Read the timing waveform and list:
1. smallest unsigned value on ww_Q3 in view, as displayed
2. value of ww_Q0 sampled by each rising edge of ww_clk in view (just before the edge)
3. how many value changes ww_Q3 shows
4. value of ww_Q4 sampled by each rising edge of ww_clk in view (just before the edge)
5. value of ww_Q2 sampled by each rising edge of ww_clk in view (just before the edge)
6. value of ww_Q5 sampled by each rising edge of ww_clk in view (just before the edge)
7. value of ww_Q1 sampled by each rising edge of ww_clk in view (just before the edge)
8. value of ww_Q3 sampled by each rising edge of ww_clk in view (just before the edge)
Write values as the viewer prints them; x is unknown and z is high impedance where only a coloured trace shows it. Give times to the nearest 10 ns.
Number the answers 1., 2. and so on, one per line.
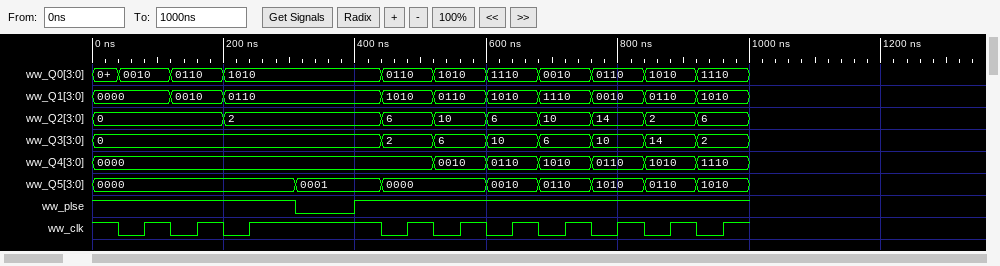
1. 0
2. 0010, 0110, 1010, 0110, 1010, 1110, 0010, 0110, 1010, 1110
3. 7
4. 0000, 0000, 0000, 0000, 0010, 0110, 1010, 0110, 1010, 1110
5. 0, 0, 2, 6, 10, 6, 10, 14, 2, 6
6. 0000, 0000, 0000, 0000, 0000, 0010, 0110, 1010, 0110, 1010
7. 0000, 0010, 0110, 1010, 0110, 1010, 1110, 0010, 0110, 1010
8. 0, 0, 0, 2, 6, 10, 6, 10, 14, 2
